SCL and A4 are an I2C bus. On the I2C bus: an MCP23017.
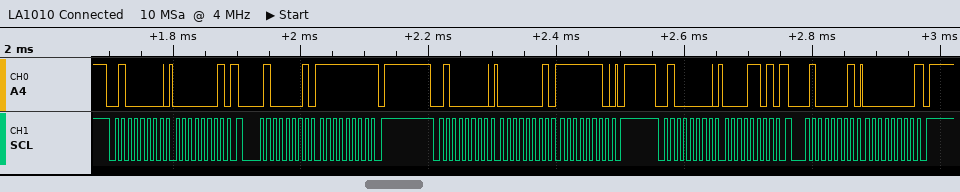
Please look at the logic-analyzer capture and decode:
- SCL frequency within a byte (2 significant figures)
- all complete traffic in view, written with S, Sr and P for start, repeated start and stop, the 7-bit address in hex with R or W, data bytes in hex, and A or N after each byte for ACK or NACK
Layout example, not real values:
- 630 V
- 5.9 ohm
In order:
- 100 kHz
- S 20W A 01 A Sr 20R A FF N P S 20W A 01 A FE A P S 20W A 0D A Sr 20R A 00 N P
